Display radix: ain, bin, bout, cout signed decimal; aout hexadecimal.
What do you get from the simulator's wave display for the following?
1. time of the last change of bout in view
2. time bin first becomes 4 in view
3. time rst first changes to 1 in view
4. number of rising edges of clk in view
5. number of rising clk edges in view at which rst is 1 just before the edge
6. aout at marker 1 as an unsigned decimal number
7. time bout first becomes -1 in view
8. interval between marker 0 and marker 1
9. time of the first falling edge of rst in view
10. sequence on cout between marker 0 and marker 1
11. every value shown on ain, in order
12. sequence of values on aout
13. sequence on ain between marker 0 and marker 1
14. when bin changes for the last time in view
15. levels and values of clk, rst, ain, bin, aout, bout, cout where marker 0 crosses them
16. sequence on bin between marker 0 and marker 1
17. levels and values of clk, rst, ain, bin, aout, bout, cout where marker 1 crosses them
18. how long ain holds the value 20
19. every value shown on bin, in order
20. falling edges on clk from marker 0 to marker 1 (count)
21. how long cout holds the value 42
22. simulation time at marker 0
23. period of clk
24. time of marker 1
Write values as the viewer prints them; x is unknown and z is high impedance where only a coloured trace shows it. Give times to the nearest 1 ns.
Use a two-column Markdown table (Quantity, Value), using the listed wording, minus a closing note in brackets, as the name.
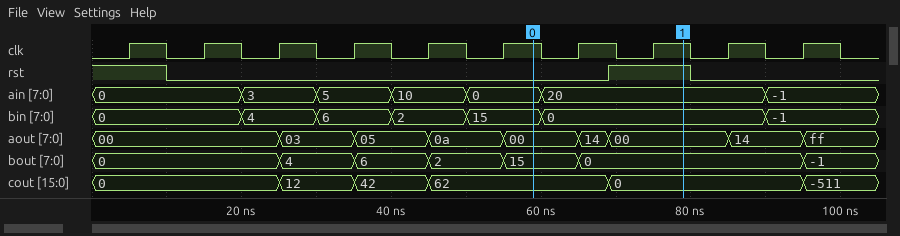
| Quantity | Value |
|---|---|
| time of the last change of bout in view | 95 ns |
| time bin first becomes 4 in view | 20 ns |
| time rst first changes to 1 in view | 69 ns |
| number of rising edges of clk in view | 10 |
| number of rising clk edges in view at which rst is 1 just before the edge | 2 |
| aout at marker 1 as an unsigned decimal number | 0 |
| time bout first becomes -1 in view | 95 ns |
| interval between marker 0 and marker 1 | 20 ns |
| time of the first falling edge of rst in view | 10 ns |
| sequence on cout between marker 0 and marker 1 | 62, 0 |
| every value shown on ain, in order | 0, 3, 5, 10, 0, 20, -1 |
| sequence of values on aout | 00, 03, 05, 0a, 00, 14, 00, 14, ff |
| sequence on ain between marker 0 and marker 1 | 0, 20 |
| when bin changes for the last time in view | 90 ns |
| levels and values of clk, rst, ain, bin, aout, bout, cout where marker 0 crosses them | clk=1, rst=0, ain=0, bin=15, aout=00, bout=15, cout=62 |
| sequence on bin between marker 0 and marker 1 | 15, 0 |
| levels and values of clk, rst, ain, bin, aout, bout, cout where marker 1 crosses them | clk=1, rst=1, ain=20, bin=0, aout=00, bout=0, cout=0 |
| how long ain holds the value 20 | 30 ns |
| every value shown on bin, in order | 0, 4, 6, 2, 15, 0, -1 |
| falling edges on clk from marker 0 to marker 1 | 2 |
| how long cout holds the value 42 | 10 ns |
| simulation time at marker 0 | 59 ns |
| period of clk | 10 ns |
| time of marker 1 | 79 ns |
